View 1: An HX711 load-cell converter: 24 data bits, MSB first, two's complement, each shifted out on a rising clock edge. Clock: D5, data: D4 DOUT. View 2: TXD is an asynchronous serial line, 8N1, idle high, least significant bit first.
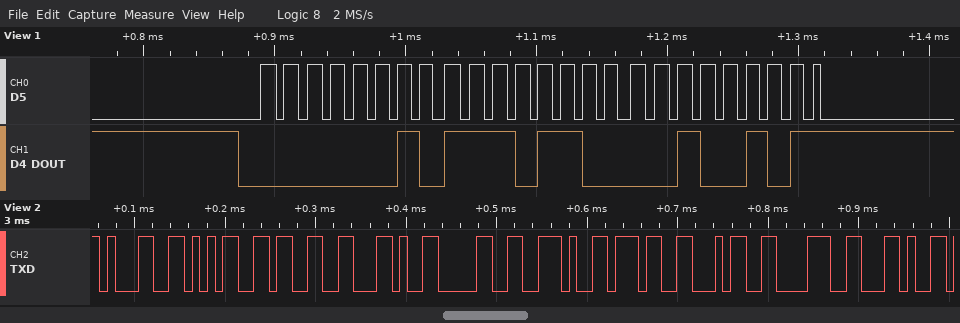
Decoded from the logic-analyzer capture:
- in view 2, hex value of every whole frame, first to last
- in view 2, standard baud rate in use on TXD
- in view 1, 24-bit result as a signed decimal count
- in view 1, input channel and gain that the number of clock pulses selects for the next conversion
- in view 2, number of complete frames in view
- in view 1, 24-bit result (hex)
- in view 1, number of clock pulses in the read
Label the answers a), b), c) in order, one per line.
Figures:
a) 0x31 0x35 0x33 0x2C 0x30 0x2E 0x37 0x34 0x38 0x2C
b) 115200 baud
c) 191525
d) channel A, gain 128
e) 10
f) 0x02EC25
g) 25
